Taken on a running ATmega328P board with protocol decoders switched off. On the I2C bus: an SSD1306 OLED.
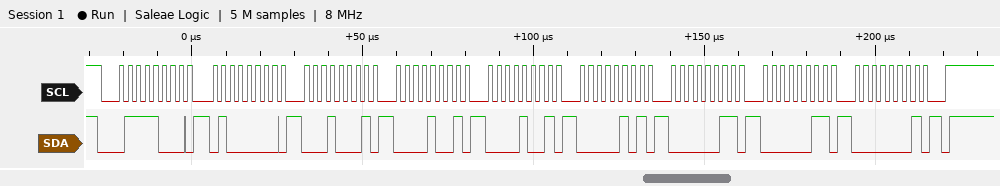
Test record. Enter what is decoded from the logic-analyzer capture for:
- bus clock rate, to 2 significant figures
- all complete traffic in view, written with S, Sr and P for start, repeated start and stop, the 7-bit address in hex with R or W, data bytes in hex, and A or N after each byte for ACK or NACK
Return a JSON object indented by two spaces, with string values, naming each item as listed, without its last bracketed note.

{
  "bus clock rate, to 2 significant figures": "400 kHz",
  "all complete traffic in view, written with S, Sr and P for start, repeated start and stop, the 7-bit address in hex with R or W, data bytes in hex, and A or N after each byte for ACK or NACK": "S 3CW A 40 A 11 A 09 A 09 A 05 A 03 A 03 A 01 A P"
}
